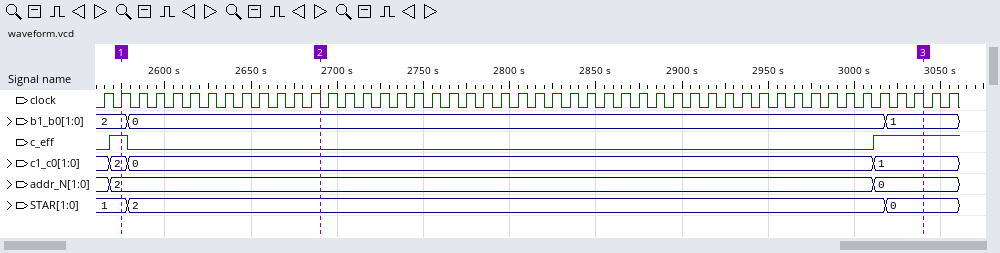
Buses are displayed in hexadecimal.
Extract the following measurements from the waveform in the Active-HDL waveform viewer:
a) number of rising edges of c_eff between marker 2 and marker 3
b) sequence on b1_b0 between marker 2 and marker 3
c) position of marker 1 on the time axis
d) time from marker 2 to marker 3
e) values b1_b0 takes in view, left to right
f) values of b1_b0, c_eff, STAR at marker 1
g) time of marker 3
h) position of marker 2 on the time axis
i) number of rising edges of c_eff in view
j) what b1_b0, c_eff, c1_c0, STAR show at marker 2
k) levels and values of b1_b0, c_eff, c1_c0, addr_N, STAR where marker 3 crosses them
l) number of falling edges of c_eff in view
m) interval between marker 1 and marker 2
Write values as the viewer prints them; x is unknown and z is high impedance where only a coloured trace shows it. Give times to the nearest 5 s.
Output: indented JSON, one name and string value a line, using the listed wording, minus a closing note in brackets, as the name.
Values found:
{
  "number of rising edges of c_eff between marker 2 and marker 3": "1",
  "sequence on b1_b0 between marker 2 and marker 3": "0, 1",
  "position of marker 1 on the time axis": "2575 s",
  "time from marker 2 to marker 3": "350 s",
  "values b1_b0 takes in view, left to right": "2, 0, 1",
  "values of b1_b0, c_eff, STAR at marker 1": "b1_b0=2, c_eff=1, STAR=1",
  "time of marker 3": "3040 s",
  "position of marker 2 on the time axis": "2690 s",
  "number of rising edges of c_eff in view": "2",
  "what b1_b0, c_eff, c1_c0, STAR show at marker 2": "b1_b0=0, c_eff=0, c1_c0=0, STAR=2",
  "levels and values of b1_b0, c_eff, c1_c0, addr_N, STAR where marker 3 crosses them": "b1_b0=1, c_eff=1, c1_c0=1, addr_N=0, STAR=0",
  "number of falling edges of c_eff in view": "1",
  "interval between marker 1 and marker 2": "115 s"
}
